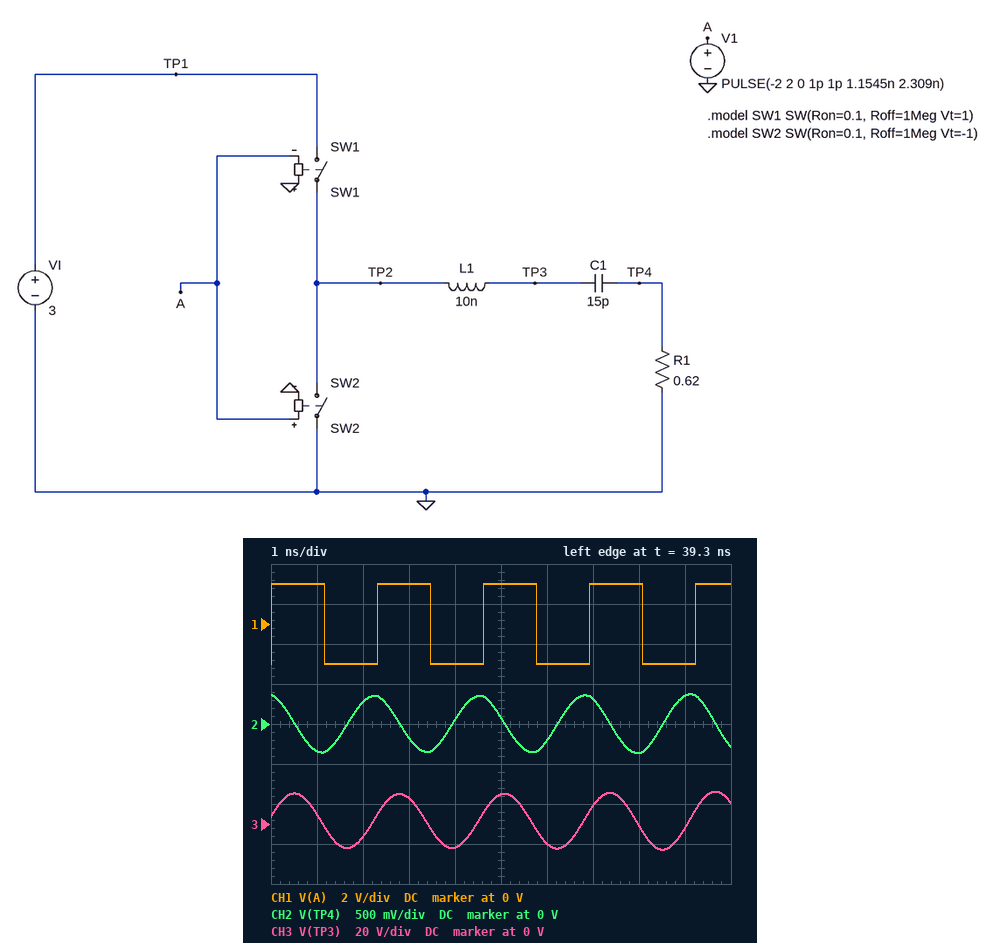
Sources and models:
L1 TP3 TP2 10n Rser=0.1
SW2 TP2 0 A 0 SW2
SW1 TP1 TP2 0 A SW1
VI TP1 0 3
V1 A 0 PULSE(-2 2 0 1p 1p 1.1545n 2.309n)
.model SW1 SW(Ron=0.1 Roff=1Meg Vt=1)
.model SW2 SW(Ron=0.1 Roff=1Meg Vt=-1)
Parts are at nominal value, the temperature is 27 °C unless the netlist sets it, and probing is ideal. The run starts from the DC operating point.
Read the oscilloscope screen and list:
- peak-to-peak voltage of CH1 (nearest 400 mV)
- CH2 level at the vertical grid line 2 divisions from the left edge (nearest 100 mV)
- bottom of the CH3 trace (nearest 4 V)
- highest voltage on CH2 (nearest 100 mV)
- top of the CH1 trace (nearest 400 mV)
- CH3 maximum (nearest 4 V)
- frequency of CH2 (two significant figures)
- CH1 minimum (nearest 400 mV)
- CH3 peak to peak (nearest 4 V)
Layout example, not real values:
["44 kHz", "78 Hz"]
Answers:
["4.0 V", "300 mV", "-12 V", "400 mV", "2.0 V", "16 V", "440 MHz", "-2.0 V", "28 V"]
